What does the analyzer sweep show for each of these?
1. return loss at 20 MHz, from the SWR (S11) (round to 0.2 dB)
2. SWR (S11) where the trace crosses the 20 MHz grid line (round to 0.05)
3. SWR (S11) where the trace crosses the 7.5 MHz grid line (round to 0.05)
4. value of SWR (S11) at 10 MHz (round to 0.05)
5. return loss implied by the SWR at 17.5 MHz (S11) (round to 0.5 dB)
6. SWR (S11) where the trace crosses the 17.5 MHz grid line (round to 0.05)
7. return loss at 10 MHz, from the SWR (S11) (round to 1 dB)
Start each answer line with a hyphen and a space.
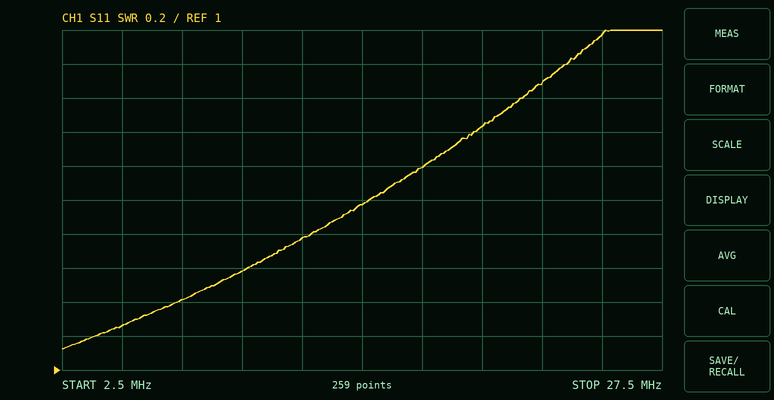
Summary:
- 7.6 dB
- 2.45
- 1.40
- 1.60
- 8.5 dB
- 2.20
- 13 dB
